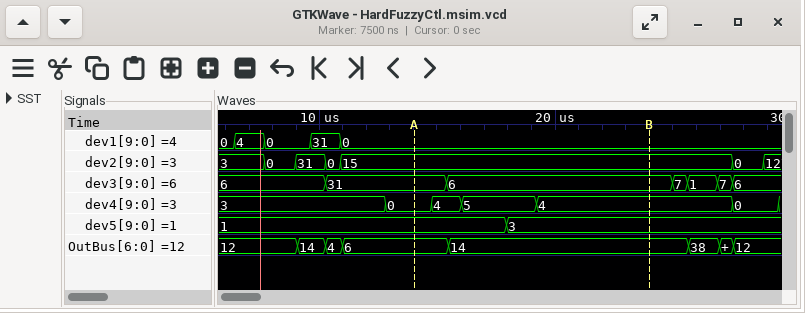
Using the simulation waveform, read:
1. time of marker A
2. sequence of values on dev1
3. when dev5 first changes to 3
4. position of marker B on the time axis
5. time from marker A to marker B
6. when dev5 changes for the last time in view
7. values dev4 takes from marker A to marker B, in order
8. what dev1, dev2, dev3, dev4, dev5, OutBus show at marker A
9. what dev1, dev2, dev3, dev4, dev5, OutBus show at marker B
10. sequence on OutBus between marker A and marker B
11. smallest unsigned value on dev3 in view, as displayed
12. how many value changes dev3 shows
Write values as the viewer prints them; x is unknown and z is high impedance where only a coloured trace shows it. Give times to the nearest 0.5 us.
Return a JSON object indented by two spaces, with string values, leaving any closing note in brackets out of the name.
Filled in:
{
  "time of marker A": "14 us",
  "sequence of values on dev1": "0, 4, 0, 31, 0",
  "when dev5 first changes to 3": "18 us",
  "position of marker B on the time axis": "24 us",
  "time from marker A to marker B": "10 us",
  "when dev5 changes for the last time in view": "18 us",
  "values dev4 takes from marker A to marker B, in order": "0, 4, 5, 4",
  "what dev1, dev2, dev3, dev4, dev5, OutBus show at marker A": "dev1=0, dev2=15, dev3=31, dev4=0, dev5=1, OutBus=6",
  "what dev1, dev2, dev3, dev4, dev5, OutBus show at marker B": "dev1=0, dev2=15, dev3=6, dev4=4, dev5=3, OutBus=14",
  "sequence on OutBus between marker A and marker B": "6, 14",
  "smallest unsigned value on dev3 in view, as displayed": "1",
  "how many value changes dev3 shows": "6"
}
